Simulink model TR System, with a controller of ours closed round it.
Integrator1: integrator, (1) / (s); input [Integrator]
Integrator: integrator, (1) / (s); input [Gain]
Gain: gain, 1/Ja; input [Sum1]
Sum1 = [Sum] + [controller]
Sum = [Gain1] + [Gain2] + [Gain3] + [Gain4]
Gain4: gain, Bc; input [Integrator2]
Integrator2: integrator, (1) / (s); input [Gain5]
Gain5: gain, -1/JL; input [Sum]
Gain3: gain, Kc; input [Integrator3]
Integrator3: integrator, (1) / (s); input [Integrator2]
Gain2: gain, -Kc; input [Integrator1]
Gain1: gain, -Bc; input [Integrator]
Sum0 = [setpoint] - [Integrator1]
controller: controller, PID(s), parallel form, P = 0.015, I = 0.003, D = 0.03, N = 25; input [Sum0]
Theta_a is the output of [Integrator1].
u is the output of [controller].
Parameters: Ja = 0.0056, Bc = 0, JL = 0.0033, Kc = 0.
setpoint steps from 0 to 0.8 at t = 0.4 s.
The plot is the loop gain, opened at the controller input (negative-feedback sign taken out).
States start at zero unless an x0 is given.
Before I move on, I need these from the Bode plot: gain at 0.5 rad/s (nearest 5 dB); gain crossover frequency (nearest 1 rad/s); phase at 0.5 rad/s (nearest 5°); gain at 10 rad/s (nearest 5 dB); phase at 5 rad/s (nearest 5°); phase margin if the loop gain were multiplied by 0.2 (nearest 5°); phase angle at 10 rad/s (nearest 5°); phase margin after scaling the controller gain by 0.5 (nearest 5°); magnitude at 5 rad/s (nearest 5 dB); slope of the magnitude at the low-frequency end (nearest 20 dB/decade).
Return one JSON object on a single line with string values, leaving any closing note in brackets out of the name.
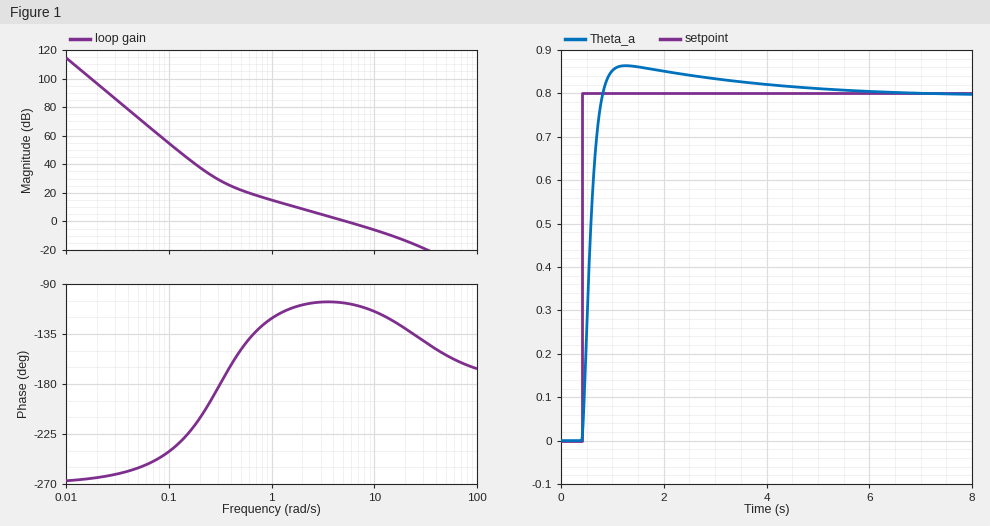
{"gain at 0.5 rad/s": "20 dB", "gain crossover frequency": "5 rad/s", "phase at 0.5 rad/s": "-150°", "gain at 10 rad/s": "-5 dB", "phase at 5 rad/s": "-105°", "phase margin if the loop gain were multiplied by 0.2": "60°", "phase angle at 10 rad/s": "-115°", "phase margin after scaling the controller gain by 0.5": "75°", "magnitude at 5 rad/s": "0 dB", "slope of the magnitude at the low-frequency end": "-60 dB/decade"}
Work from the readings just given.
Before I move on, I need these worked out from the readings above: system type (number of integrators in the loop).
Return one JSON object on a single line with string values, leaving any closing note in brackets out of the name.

{"system type": "3"}
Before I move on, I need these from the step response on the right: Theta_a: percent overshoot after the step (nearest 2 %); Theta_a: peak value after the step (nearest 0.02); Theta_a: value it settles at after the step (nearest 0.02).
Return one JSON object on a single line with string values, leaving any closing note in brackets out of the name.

{"Theta_a: percent overshoot after the step": "8 %", "Theta_a: peak value after the step": "0.86", "Theta_a: value it settles at after the step": "0.80"}
